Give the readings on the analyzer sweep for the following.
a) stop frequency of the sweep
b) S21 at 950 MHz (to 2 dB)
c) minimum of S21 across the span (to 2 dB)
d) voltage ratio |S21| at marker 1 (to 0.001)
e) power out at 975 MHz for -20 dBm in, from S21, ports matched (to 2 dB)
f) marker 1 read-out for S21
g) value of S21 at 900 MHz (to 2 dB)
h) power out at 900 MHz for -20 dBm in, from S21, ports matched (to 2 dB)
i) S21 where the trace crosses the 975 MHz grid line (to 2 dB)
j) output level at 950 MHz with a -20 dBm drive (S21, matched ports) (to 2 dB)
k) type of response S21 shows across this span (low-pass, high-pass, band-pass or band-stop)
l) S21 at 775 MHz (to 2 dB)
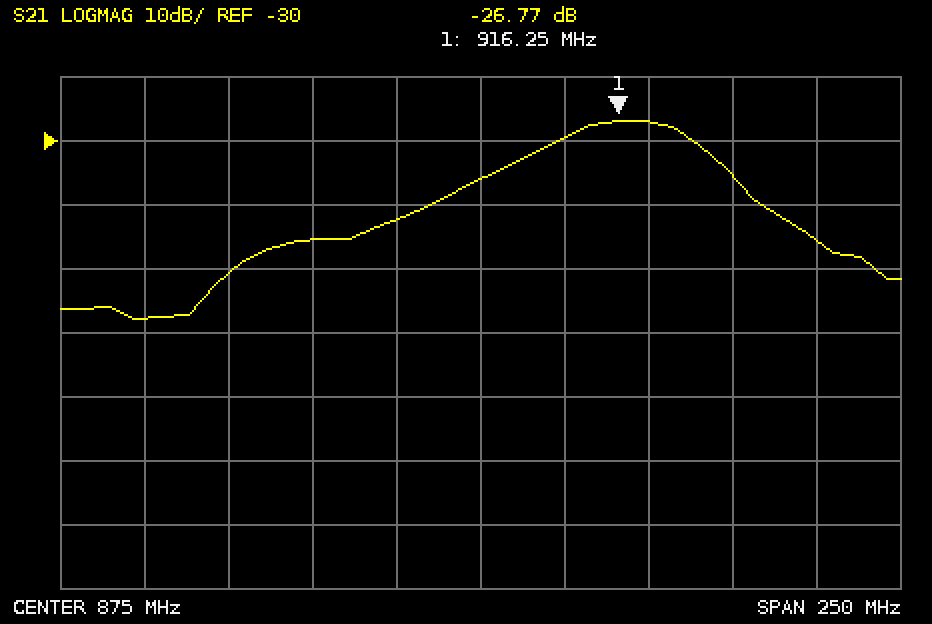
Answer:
1 GHz
-36 dB
-58 dB
0.046
-66 dBm
-26.77 dB
-30 dB
-50 dBm
-46 dB
-56 dBm
band-pass
-58 dB
